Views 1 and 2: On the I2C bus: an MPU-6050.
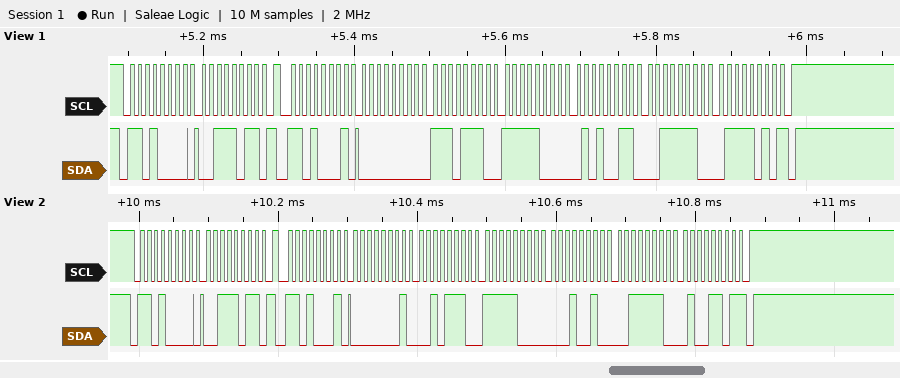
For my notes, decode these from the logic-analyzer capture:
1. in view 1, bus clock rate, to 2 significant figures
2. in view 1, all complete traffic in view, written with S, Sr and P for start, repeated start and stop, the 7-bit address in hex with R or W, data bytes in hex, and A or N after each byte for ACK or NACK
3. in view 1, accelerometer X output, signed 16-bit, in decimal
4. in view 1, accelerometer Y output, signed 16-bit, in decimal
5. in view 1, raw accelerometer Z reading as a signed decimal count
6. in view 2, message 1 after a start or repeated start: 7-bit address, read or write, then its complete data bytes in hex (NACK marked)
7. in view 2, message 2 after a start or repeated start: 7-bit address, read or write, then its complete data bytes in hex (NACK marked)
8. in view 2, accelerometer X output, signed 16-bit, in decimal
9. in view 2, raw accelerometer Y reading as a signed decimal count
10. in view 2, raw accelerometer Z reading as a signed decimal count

100 kHz
S 68W A 3B A Sr 68R A 00 A EE A F8 A 53 A 3E A 7A N P
238
-1965
15994
0x68 write: 3B
0x68 read: 01 2E F8 12 3E 4D NACK
302
-2030
15949
